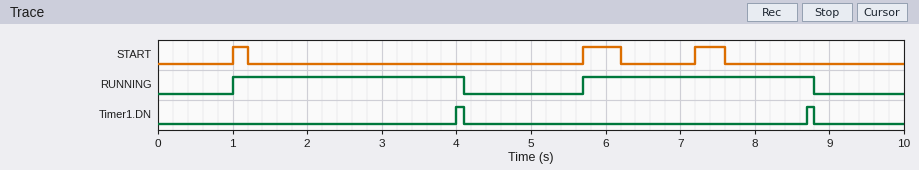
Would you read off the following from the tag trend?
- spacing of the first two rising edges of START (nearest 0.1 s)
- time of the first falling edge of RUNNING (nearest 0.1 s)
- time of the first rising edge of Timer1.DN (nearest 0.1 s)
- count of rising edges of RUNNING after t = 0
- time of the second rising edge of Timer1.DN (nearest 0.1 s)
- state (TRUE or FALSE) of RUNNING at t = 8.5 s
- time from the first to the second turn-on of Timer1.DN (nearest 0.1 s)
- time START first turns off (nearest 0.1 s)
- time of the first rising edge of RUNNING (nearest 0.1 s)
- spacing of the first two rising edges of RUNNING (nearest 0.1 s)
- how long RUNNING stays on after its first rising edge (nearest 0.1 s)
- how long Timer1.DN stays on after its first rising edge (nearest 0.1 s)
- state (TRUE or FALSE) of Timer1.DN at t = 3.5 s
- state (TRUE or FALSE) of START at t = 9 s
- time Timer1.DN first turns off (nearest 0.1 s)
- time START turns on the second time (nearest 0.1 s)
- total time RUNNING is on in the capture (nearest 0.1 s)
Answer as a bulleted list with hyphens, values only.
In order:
- 4.7 s
- 4.1 s
- 4.0 s
- 2
- 8.7 s
- TRUE
- 4.7 s
- 1.2 s
- 1.0 s
- 4.7 s
- 3.1 s
- 0.1 s
- FALSE
- FALSE
- 4.1 s
- 5.7 s
- 6.2 s
